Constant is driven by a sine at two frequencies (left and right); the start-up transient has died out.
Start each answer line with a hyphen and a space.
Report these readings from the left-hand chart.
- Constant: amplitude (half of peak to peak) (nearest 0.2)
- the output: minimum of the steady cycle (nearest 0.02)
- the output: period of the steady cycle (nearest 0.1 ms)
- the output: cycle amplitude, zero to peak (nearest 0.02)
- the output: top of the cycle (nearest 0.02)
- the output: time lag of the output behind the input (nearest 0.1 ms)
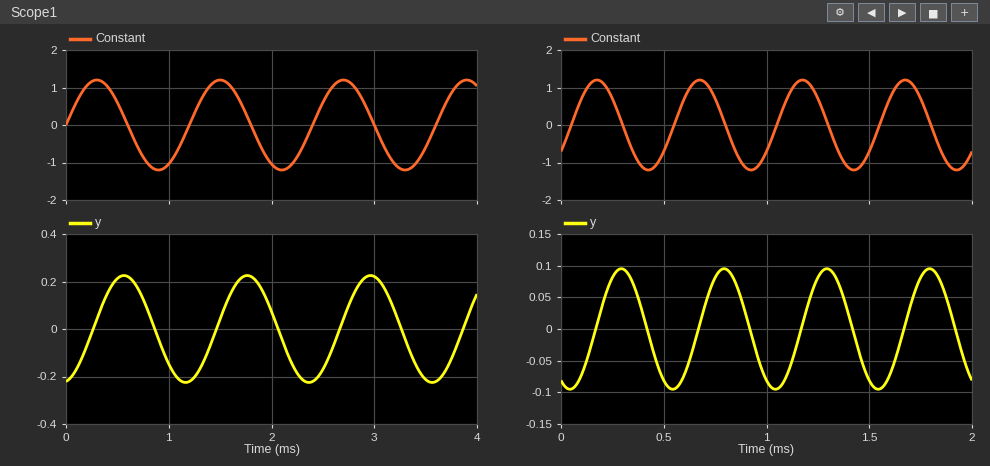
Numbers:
- 1.2
- -0.22
- 1.2 ms
- 0.22
- 0.22
- 0.3 ms
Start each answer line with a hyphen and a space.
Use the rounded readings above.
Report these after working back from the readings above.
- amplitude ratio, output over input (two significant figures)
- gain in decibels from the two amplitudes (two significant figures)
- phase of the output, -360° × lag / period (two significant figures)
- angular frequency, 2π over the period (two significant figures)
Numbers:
- 0.18
- -15 dB
- -90°
- 5.2 rad/ms
